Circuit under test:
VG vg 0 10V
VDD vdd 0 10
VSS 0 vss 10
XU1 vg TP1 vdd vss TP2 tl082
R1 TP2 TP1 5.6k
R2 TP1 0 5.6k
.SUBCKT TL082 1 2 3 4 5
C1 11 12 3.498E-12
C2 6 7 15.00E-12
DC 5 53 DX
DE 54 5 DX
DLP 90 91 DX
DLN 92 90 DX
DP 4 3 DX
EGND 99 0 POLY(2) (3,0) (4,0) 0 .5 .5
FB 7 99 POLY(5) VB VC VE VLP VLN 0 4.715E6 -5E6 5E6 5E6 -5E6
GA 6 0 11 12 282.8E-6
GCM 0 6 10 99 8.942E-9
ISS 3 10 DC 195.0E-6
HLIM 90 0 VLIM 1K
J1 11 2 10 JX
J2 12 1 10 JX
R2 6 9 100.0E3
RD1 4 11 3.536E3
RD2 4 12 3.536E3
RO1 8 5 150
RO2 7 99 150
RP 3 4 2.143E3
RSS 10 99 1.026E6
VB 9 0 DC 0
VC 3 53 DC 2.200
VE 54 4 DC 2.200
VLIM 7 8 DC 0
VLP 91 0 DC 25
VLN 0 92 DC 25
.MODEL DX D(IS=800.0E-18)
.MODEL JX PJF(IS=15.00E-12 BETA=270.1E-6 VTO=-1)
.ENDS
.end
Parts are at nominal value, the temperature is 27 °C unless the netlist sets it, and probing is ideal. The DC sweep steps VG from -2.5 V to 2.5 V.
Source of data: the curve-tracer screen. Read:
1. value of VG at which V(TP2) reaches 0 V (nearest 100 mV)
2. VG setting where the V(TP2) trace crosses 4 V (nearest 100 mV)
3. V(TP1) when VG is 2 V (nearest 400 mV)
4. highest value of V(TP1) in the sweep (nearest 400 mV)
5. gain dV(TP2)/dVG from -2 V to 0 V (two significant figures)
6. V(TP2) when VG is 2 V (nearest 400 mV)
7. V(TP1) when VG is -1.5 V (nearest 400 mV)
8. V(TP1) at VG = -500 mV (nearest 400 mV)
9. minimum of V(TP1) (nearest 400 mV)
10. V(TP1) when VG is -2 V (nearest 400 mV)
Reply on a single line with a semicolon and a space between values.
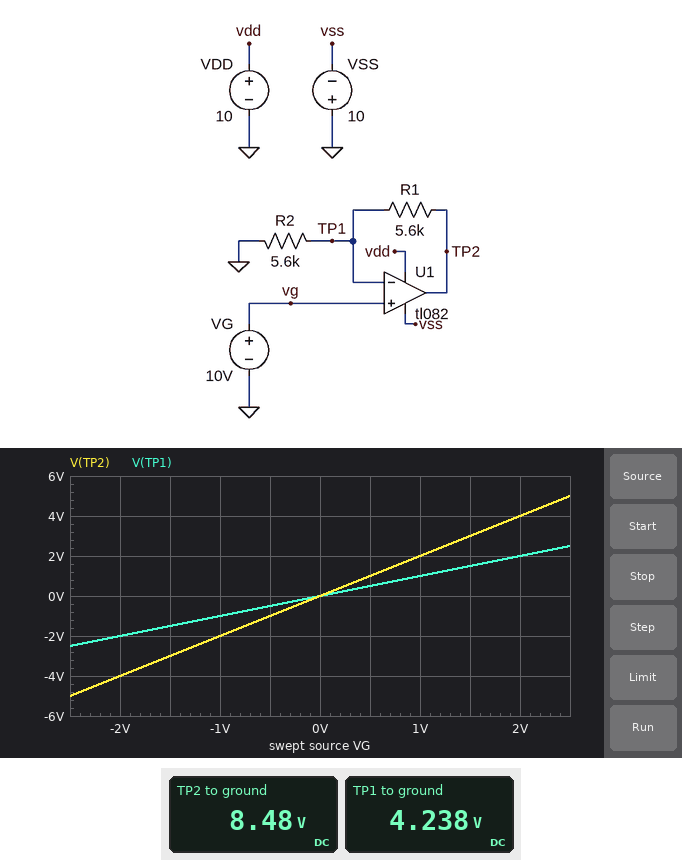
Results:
0 V; 2.0 V; 2.0 V; 2.4 V; 2.0 V/V; 4.0 V; -1.6 V; -400 mV; -2.4 V; -2.0 V
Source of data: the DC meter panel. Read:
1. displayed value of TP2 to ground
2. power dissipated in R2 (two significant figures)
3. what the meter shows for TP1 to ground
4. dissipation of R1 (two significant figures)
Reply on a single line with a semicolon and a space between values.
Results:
8.48 V; 3.2 mW; 4.238 V; 3.2 mW
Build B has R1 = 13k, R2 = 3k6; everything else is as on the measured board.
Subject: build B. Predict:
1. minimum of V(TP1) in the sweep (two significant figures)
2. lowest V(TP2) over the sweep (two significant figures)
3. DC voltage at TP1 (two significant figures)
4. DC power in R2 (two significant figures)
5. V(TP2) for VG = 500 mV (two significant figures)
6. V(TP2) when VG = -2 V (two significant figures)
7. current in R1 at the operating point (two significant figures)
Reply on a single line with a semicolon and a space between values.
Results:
-1.8 V; -8.5 V; 1.8 V; 940 µW; 2.3 V; -8.4 V; 510 µA
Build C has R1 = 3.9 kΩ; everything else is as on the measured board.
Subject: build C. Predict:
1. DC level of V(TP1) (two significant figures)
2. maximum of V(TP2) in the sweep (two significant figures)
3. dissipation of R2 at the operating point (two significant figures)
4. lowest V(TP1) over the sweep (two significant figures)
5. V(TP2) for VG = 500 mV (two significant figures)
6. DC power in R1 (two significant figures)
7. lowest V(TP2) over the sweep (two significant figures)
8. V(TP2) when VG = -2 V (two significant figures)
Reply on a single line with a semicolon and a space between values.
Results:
5.0 V; 4.2 V; 4.5 mW; -2.5 V; 850 mV; 3.1 mW; -4.2 V; -3.4 V
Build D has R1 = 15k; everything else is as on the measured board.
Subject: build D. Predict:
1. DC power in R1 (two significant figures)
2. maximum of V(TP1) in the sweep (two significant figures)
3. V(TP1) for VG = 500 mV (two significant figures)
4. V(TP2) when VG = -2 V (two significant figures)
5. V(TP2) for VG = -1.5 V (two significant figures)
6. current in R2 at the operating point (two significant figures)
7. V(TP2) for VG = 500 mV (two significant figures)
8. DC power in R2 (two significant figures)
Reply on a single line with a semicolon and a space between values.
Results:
2.5 mW; 2.3 V; 500 mV; -7.4 V; -5.5 V; 410 µA; 1.8 V; 950 µW
